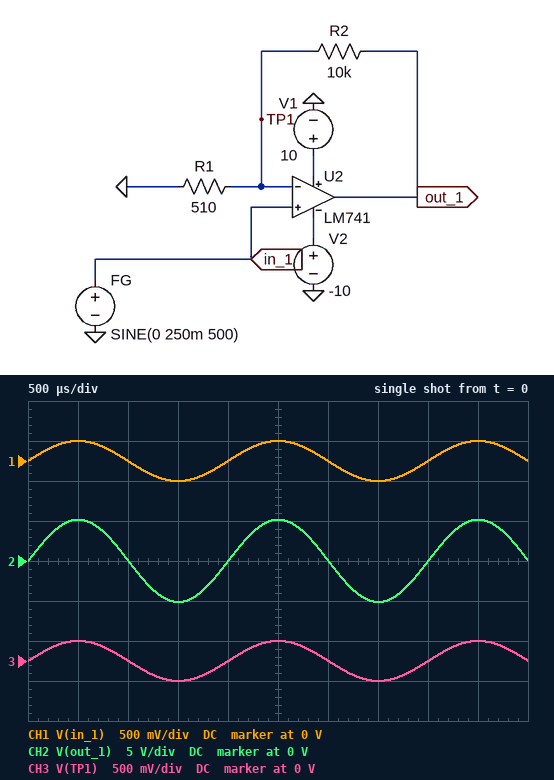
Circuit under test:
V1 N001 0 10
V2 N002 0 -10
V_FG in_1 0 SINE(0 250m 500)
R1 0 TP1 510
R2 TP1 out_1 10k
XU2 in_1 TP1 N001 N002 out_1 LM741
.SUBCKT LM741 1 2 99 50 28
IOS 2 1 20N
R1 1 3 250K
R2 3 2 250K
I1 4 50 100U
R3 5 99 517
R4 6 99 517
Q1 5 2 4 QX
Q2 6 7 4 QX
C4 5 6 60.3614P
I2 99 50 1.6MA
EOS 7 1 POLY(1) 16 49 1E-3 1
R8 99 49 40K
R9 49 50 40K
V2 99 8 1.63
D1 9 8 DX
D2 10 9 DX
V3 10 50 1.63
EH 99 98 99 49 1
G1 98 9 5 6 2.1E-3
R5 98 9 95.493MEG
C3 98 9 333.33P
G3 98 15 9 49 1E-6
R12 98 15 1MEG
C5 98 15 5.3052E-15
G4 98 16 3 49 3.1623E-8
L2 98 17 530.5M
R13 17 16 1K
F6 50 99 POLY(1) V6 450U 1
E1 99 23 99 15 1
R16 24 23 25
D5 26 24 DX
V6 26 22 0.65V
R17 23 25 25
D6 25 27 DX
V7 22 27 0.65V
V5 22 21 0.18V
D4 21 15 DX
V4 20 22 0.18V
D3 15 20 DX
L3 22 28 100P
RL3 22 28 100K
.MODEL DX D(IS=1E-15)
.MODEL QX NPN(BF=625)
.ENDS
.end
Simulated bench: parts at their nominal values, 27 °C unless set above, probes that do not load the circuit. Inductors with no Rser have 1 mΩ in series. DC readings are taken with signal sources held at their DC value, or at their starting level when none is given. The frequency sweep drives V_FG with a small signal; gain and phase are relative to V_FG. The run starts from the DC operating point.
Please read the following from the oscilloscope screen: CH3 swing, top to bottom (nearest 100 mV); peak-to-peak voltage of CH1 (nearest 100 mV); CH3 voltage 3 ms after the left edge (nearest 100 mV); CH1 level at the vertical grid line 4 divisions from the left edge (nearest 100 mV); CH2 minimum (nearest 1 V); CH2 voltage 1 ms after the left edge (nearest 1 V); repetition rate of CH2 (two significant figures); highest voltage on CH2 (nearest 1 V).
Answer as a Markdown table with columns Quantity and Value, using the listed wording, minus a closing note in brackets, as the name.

| Quantity | Value |
|---|---|
| CH3 swing, top to bottom | 500 mV |
| peak-to-peak voltage of CH1 | 500 mV |
| CH3 voltage 3 ms after the left edge | 0 V |
| CH1 level at the vertical grid line 4 divisions from the left edge | 0 V |
| CH2 minimum | -5 V |
| CH2 voltage 1 ms after the left edge | 0 V |
| repetition rate of CH2 | 500 Hz |
| highest voltage on CH2 | 5 V |
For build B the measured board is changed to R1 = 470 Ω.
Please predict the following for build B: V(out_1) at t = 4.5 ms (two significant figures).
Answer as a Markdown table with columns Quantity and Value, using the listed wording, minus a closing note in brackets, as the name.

| Quantity | Value |
|---|---|
| V(out_1) at t = 4.5 ms | 5.6 V |
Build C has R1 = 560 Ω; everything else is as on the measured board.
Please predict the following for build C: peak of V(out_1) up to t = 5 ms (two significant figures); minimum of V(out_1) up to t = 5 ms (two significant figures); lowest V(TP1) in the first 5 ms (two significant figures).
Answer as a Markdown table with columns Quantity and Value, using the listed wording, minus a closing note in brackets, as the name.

| Quantity | Value |
|---|---|
| peak of V(out_1) up to t = 5 ms | 4.7 V |
| minimum of V(out_1) up to t = 5 ms | -4.7 V |
| lowest V(TP1) in the first 5 ms | -250 mV |
